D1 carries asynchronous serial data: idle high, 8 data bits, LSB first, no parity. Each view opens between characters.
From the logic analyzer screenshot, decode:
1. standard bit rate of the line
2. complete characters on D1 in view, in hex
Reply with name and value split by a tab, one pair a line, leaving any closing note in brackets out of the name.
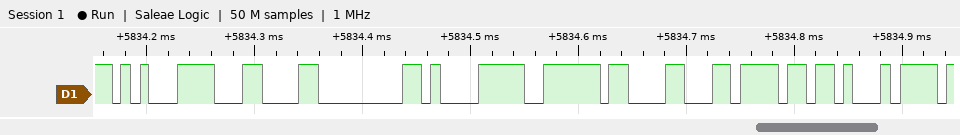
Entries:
standard bit rate of the line	115200 baud
complete characters on D1 in view, in hex	C5, 0C, 00, E1, 7E, 18, 6F, D1
